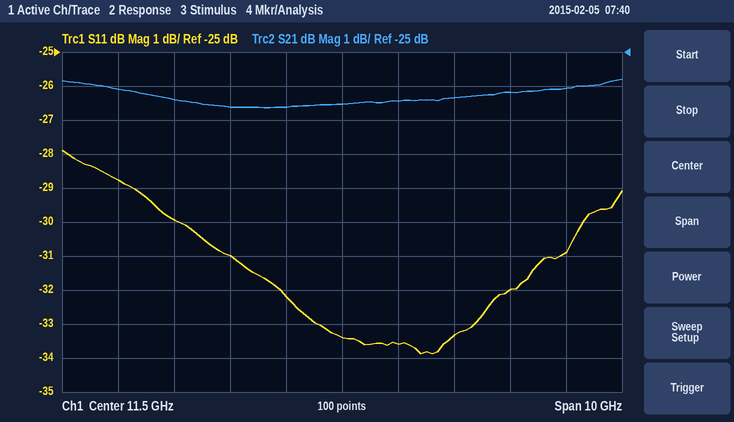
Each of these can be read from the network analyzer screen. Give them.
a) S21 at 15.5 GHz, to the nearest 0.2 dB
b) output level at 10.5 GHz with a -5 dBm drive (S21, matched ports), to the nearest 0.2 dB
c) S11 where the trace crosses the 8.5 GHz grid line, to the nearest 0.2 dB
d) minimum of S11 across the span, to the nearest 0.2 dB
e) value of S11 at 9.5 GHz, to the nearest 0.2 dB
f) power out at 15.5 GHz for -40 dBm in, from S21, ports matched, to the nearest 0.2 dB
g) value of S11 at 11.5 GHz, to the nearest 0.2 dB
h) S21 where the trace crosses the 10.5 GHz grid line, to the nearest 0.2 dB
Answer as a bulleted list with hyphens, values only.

- -26.0 dB
- -31.6 dBm
- -30.0 dB
- -33.8 dB
- -31.0 dB
- -66.0 dBm
- -33.4 dB
- -26.6 dB
